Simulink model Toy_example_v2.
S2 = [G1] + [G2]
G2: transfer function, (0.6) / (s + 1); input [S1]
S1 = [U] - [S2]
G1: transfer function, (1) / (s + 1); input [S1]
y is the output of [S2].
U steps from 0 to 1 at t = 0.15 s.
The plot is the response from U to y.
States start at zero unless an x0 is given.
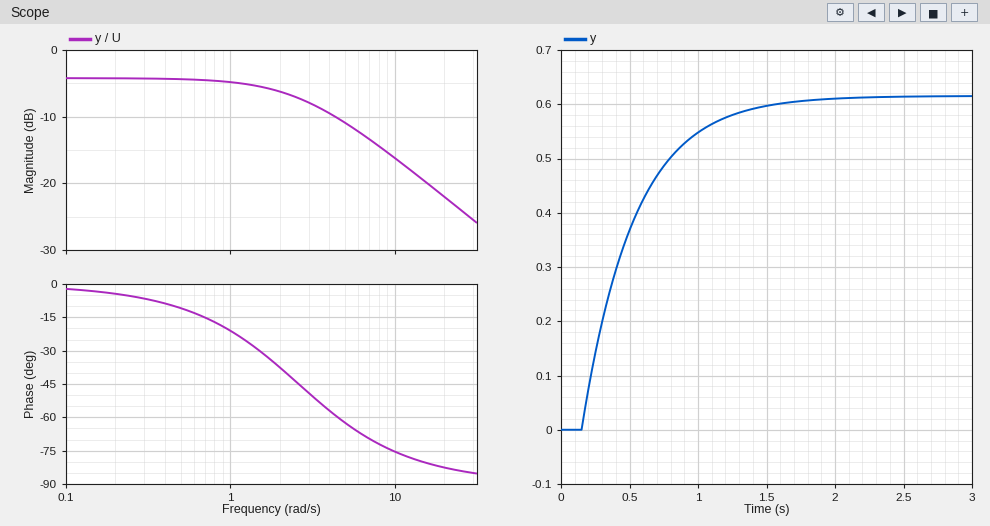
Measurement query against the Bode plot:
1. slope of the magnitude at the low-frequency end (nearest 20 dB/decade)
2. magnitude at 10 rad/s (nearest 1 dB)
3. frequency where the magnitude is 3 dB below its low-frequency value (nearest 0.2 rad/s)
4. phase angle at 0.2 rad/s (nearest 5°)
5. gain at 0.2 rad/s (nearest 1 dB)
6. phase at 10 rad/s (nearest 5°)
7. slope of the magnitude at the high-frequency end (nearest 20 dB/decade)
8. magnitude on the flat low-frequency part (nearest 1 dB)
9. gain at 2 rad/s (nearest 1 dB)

0 dB/decade
-16 dB
2.6 rad/s
-5°
-4 dB
-75°
-20 dB/decade
-4 dB
-6 dB
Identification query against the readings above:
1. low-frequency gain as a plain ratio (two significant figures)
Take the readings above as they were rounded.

0.63
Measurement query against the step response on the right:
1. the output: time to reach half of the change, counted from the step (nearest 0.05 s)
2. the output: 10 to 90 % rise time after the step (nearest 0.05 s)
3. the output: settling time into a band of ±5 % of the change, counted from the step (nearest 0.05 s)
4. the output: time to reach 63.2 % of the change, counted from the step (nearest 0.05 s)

0.25 s
0.85 s
1.15 s
0.40 s
